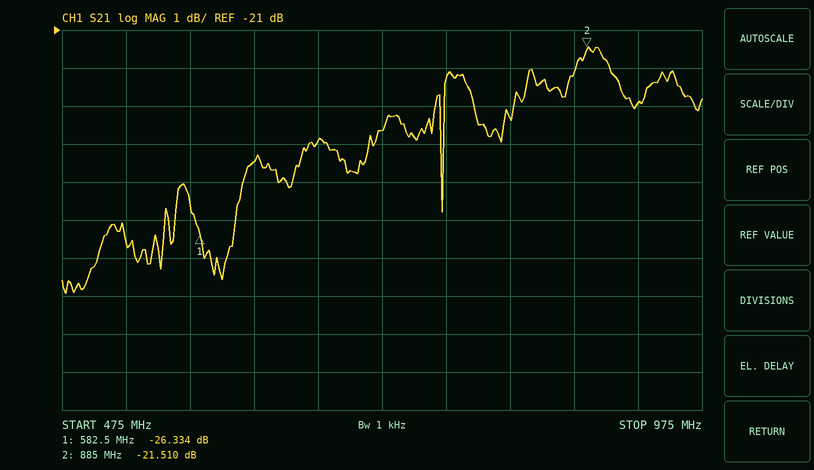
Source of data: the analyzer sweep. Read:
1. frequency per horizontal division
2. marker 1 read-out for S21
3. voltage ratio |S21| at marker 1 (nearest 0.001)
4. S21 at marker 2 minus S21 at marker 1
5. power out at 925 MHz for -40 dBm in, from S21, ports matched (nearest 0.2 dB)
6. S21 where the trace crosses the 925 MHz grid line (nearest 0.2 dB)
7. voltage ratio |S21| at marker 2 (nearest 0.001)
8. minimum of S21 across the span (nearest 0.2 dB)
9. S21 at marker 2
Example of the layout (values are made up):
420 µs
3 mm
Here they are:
50 MHz
-26.334 dB
0.048
4.824 dB
-63.0 dBm
-23.0 dB
0.084
-28.0 dB
-21.510 dB
